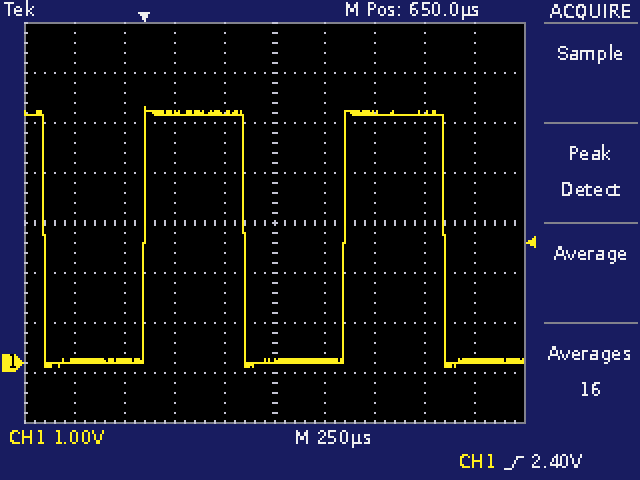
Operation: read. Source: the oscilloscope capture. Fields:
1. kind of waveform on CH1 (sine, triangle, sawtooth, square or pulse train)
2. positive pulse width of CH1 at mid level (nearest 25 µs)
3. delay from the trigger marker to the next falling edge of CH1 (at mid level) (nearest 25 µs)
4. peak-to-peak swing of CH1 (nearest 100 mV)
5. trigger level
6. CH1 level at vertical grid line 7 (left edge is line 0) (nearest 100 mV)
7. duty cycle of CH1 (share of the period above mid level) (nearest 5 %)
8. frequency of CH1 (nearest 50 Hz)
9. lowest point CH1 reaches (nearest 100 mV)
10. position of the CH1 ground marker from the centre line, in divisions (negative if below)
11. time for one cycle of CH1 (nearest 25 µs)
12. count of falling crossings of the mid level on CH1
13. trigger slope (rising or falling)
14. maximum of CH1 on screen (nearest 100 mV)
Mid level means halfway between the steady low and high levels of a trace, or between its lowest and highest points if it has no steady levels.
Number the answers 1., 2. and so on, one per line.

1. square
2. 500 µs
3. 500 µs
4. 5.2 V
5. 2.40 V
6. 5.0 V
7. 50 %
8. 1.00 kHz
9. -100 mV
10. -2.8 div
11. 1.000 ms
12. 3
13. rising
14. 5.1 V
